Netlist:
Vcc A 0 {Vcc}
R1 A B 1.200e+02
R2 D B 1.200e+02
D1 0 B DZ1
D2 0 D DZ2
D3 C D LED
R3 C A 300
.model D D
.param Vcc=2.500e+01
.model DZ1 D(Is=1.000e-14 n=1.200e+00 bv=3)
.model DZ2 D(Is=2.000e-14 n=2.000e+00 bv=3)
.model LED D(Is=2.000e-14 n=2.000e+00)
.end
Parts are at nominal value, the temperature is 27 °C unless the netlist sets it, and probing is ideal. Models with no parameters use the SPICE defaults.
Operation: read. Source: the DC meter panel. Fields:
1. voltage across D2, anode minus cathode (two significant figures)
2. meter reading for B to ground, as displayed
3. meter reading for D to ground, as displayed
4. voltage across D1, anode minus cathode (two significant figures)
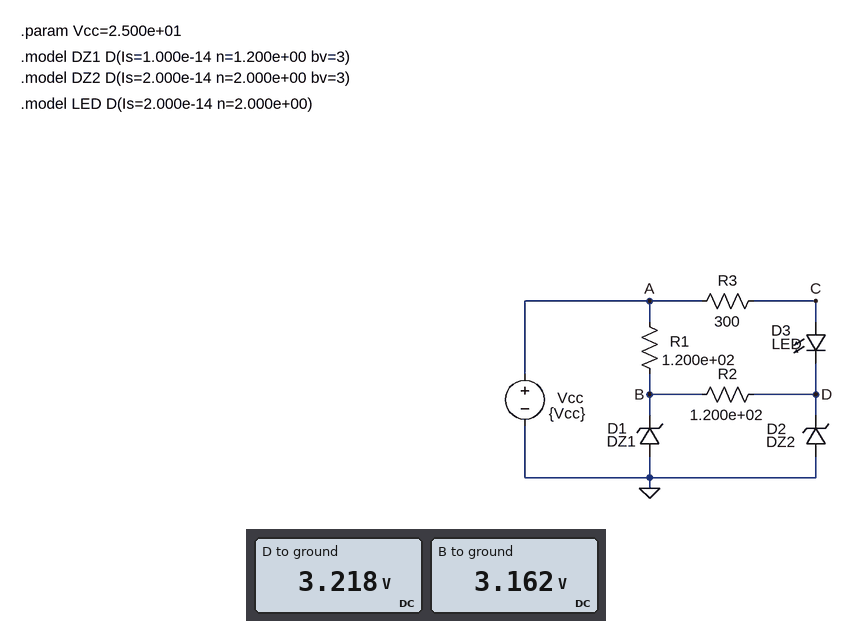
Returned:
-3.2 V
3.162 V
3.218 V
-3.2 V
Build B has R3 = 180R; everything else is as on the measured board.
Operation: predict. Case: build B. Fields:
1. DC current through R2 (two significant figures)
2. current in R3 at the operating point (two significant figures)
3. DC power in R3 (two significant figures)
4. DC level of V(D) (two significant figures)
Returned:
690 µA
110 mA
2.3 W
3.2 V
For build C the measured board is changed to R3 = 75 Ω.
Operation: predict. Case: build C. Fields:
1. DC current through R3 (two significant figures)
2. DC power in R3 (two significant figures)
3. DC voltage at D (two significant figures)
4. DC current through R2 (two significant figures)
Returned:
270 mA
5.4 W
3.3 V
1.1 mA
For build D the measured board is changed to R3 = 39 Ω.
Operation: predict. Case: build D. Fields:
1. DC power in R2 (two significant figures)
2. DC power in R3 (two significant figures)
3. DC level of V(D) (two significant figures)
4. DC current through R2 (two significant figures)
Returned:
220 µW
10 W
3.3 V
1.3 mA
